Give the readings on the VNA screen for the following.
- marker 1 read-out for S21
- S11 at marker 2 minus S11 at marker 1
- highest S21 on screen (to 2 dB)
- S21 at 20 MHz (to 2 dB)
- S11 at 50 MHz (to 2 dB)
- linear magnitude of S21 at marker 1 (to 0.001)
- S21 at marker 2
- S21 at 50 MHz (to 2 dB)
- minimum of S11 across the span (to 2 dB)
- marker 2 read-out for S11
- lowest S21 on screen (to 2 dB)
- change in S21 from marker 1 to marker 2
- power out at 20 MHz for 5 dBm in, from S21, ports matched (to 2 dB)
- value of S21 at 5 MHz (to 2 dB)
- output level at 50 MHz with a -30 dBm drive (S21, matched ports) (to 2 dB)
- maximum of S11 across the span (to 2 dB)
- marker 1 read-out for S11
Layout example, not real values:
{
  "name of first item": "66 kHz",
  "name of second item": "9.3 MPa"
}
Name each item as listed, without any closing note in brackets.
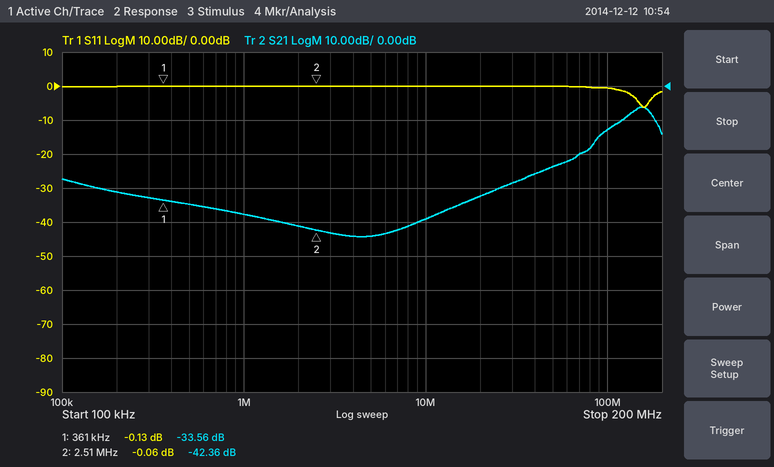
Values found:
{
  "marker 1 read-out for S21": "-33.56 dB",
  "S11 at marker 2 minus S11 at marker 1": "0.07 dB",
  "highest S21 on screen": "-6 dB",
  "S21 at 20 MHz": "-32 dB",
  "S11 at 50 MHz": "0 dB",
  "linear magnitude of S21 at marker 1": "0.021",
  "S21 at marker 2": "-42.36 dB",
  "S21 at 50 MHz": "-24 dB",
  "minimum of S11 across the span": "-6 dB",
  "marker 2 read-out for S11": "-0.06 dB",
  "lowest S21 on screen": "-44 dB",
  "change in S21 from marker 1 to marker 2": "-8.80 dB",
  "power out at 20 MHz for 5 dBm in, from S21, ports matched": "-28 dBm",
  "value of S21 at 5 MHz": "-44 dB",
  "output level at 50 MHz with a -30 dBm drive (S21, matched ports)": "-54 dBm",
  "maximum of S11 across the span": "0 dB",
  "marker 1 read-out for S11": "-0.13 dB"
}
